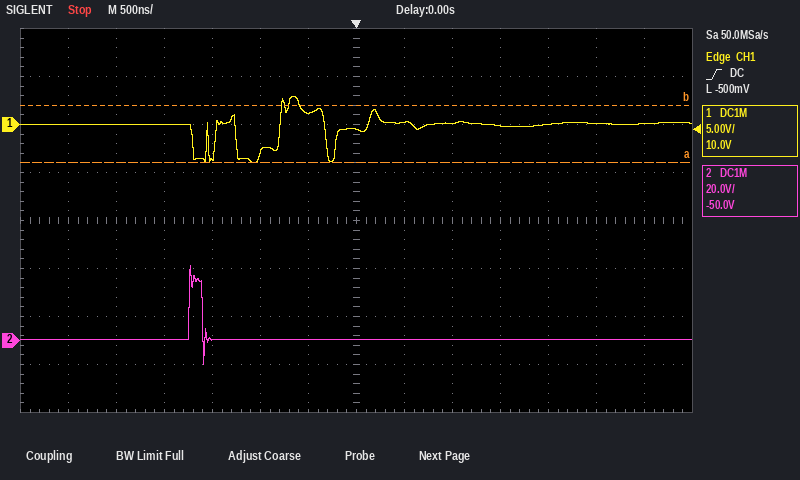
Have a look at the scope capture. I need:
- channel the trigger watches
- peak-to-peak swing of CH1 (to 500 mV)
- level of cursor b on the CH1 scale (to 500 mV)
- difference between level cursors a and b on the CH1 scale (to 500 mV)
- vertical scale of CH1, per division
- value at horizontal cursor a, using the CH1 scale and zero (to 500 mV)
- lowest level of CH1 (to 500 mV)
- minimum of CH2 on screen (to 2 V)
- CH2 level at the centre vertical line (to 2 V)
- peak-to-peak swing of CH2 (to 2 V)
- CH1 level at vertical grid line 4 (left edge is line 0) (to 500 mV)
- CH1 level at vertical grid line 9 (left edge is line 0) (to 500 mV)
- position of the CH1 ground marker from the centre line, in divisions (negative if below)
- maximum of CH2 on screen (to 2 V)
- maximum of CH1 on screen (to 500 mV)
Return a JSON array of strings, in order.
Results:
["CH1", "7.0 V", "2.0 V", "6.0 V", "5 V", "-4.0 V", "-4.0 V", "-10 V", "0 V", "42 V", "-3.5 V", "0.0 V", "+2.0 div", "32 V", "3.0 V"]
